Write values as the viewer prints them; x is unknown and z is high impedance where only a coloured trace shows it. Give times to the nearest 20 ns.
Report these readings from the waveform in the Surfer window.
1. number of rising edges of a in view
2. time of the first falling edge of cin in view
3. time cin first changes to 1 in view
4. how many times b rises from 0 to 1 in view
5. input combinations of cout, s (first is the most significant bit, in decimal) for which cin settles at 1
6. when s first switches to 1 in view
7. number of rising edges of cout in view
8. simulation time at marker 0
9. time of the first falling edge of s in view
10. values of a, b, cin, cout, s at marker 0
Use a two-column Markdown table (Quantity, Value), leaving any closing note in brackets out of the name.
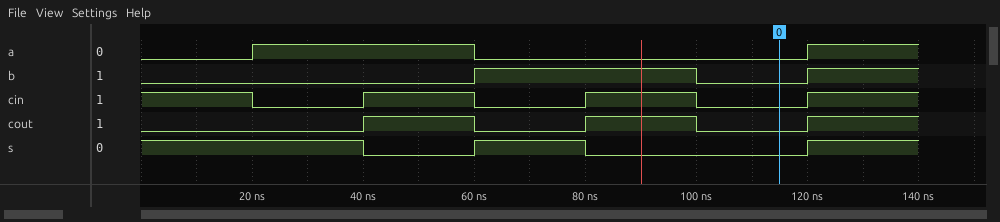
| Quantity | Value |
|---|---|
| number of rising edges of a in view | 2 |
| time of the first falling edge of cin in view | 20 ns |
| time cin first changes to 1 in view | 40 ns |
| how many times b rises from 0 to 1 in view | 2 |
| input combinations of cout, s (first is the most significant bit, in decimal) for which cin settles at 1 | 2, 3 |
| when s first switches to 1 in view | 60 ns |
| number of rising edges of cout in view | 3 |
| simulation time at marker 0 | 120 ns |
| time of the first falling edge of s in view | 40 ns |
| values of a, b, cin, cout, s at marker 0 | a=0, b=0, cin=0, cout=0, s=0 |
